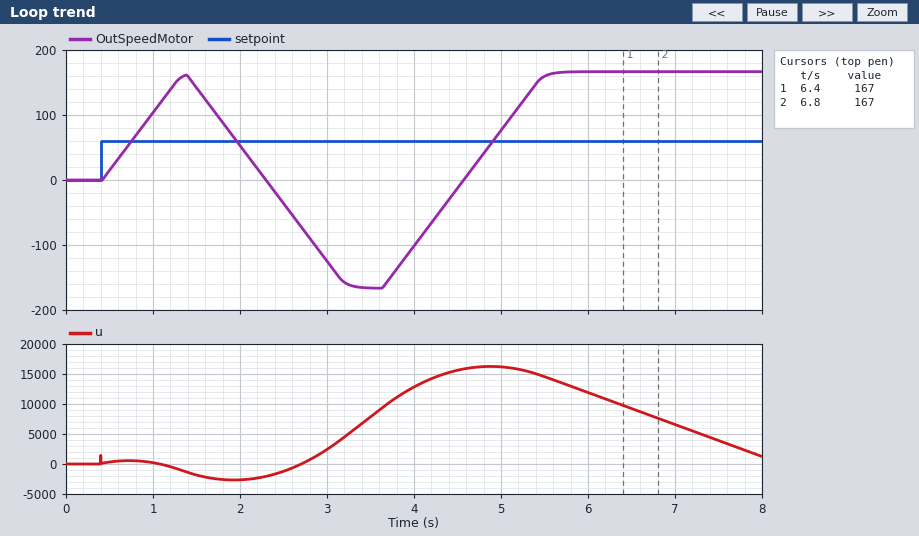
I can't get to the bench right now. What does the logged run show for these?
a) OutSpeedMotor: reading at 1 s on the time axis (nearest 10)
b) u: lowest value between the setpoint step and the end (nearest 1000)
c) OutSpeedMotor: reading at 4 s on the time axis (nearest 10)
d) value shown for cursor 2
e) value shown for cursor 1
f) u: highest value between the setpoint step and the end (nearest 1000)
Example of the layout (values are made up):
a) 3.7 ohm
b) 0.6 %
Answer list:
a) 100
b) -3000
c) -100
d) 167
e) 167
f) 16000
